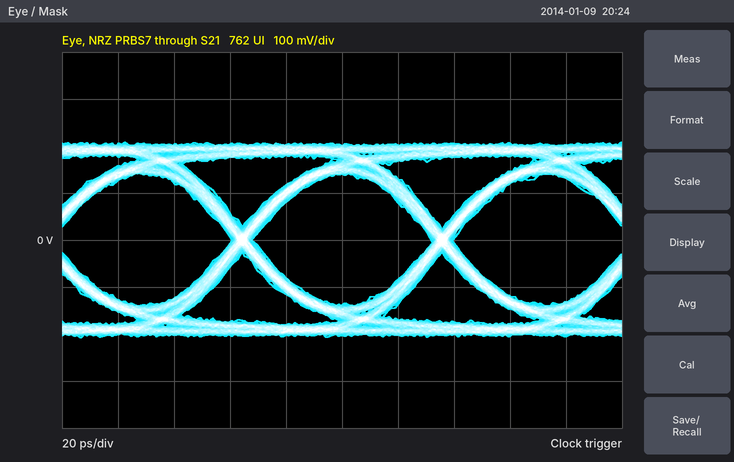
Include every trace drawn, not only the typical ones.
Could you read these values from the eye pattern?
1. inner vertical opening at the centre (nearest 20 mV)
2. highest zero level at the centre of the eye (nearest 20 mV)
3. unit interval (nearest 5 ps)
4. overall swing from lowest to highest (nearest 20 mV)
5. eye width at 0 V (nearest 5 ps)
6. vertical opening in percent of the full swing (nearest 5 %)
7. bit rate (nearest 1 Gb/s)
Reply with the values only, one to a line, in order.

280 mV
-140 mV
70 ps
420 mV
65 ps
65 %
14 Gb/s
